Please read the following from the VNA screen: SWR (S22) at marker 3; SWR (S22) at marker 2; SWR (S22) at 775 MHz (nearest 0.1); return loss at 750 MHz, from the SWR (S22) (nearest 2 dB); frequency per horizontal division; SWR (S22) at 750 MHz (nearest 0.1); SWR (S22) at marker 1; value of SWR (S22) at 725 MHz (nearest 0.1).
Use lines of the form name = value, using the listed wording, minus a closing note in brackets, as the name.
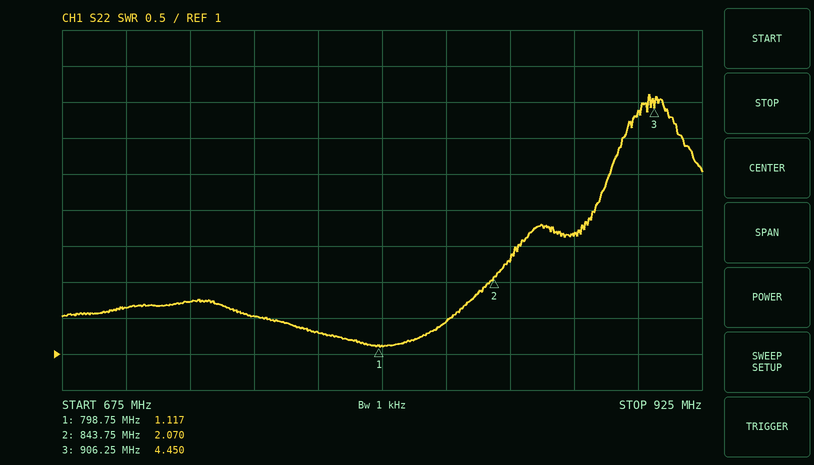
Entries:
SWR (S22) at marker 3 = 4.450
SWR (S22) at marker 2 = 2.070
SWR (S22) at 775 MHz = 1.3
return loss at 750 MHz, from the SWR (S22) = 14 dB
frequency per horizontal division = 25 MHz
SWR (S22) at 750 MHz = 1.5
SWR (S22) at marker 1 = 1.117
value of SWR (S22) at 725 MHz = 1.7
